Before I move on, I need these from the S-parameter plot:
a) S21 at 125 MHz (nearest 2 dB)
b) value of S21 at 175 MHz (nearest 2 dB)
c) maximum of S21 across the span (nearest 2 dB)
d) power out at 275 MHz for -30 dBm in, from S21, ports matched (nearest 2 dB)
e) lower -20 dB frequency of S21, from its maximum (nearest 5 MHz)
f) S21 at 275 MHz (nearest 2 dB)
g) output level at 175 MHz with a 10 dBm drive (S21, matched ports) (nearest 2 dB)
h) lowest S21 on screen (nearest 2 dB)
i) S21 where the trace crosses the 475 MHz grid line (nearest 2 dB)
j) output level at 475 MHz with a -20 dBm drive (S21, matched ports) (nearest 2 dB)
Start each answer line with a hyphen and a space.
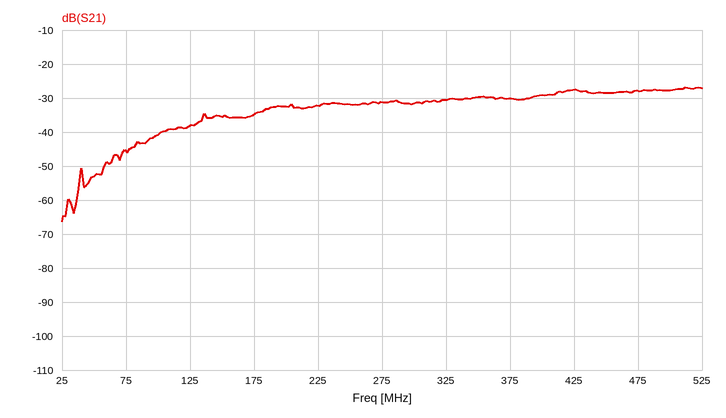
- -38 dB
- -34 dB
- -26 dB
- -62 dBm
- 70 MHz
- -32 dB
- -24 dBm
- -66 dB
- -28 dB
- -48 dBm
